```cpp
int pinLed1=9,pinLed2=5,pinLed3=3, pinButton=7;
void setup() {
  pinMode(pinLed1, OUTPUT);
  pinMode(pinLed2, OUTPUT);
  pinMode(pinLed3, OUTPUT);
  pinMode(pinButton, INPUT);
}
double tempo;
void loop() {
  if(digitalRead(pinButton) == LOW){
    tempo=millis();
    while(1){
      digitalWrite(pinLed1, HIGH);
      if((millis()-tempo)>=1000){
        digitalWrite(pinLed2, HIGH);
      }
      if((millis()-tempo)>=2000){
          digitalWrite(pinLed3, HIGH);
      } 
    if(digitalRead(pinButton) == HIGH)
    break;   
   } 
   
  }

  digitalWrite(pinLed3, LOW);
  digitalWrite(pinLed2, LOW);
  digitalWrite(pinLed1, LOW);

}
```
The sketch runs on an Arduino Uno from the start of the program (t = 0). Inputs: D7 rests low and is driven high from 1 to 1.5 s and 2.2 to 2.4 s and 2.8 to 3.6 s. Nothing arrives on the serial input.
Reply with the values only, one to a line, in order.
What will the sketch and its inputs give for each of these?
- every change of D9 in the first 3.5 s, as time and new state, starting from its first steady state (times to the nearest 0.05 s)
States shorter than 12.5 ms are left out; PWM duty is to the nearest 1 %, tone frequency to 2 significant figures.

0 s high; 1 s low; 1.5 s high; 2.2 s low; 2.4 s high; 2.8 s low
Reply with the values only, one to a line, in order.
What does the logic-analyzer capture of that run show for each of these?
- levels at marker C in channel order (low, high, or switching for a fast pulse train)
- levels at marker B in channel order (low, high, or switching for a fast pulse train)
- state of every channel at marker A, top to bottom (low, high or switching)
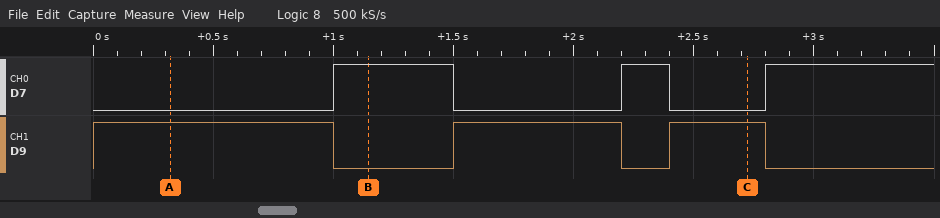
D7 low, D9 high
D7 high, D9 low
D7 low, D9 high
